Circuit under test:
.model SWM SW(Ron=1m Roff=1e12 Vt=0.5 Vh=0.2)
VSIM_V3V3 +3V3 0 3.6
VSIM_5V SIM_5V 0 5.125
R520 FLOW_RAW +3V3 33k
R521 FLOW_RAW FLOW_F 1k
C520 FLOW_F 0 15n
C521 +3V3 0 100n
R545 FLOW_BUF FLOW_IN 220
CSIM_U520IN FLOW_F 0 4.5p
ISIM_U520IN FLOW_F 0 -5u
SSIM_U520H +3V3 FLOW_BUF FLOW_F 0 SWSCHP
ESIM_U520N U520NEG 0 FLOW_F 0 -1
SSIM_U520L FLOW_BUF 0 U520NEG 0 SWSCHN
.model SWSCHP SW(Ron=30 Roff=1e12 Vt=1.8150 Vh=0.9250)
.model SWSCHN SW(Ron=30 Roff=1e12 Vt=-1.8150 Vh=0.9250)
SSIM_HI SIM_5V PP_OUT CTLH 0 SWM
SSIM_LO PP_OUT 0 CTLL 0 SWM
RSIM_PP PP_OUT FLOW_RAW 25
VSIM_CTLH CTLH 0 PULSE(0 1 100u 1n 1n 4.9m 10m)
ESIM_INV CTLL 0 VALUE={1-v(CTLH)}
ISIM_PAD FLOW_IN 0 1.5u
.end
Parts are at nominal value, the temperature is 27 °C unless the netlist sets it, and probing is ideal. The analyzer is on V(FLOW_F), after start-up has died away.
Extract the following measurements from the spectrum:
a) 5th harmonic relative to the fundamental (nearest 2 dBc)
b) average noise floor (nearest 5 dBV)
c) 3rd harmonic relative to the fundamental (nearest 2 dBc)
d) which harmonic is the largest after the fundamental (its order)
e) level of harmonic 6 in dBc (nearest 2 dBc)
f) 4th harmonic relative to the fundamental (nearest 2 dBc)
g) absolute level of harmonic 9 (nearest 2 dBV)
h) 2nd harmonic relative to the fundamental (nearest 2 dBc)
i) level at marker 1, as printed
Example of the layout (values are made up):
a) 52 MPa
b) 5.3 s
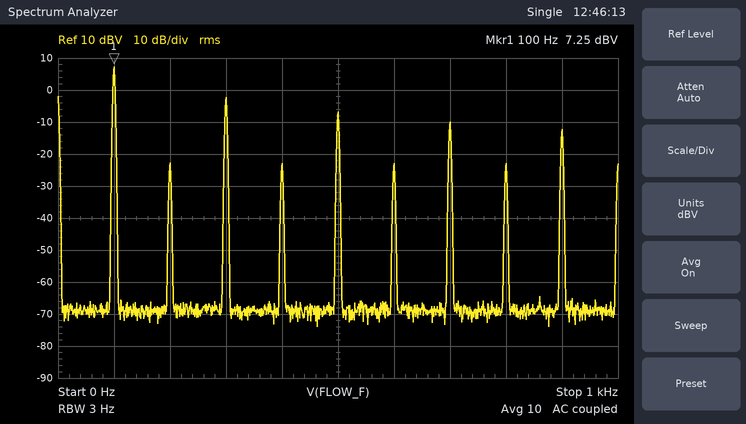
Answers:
a) -14 dBc
b) -70 dBV
c) -10 dBc
d) 3
e) -30 dBc
f) -30 dBc
g) -12 dBV
h) -30 dBc
i) 7.25 dBV
